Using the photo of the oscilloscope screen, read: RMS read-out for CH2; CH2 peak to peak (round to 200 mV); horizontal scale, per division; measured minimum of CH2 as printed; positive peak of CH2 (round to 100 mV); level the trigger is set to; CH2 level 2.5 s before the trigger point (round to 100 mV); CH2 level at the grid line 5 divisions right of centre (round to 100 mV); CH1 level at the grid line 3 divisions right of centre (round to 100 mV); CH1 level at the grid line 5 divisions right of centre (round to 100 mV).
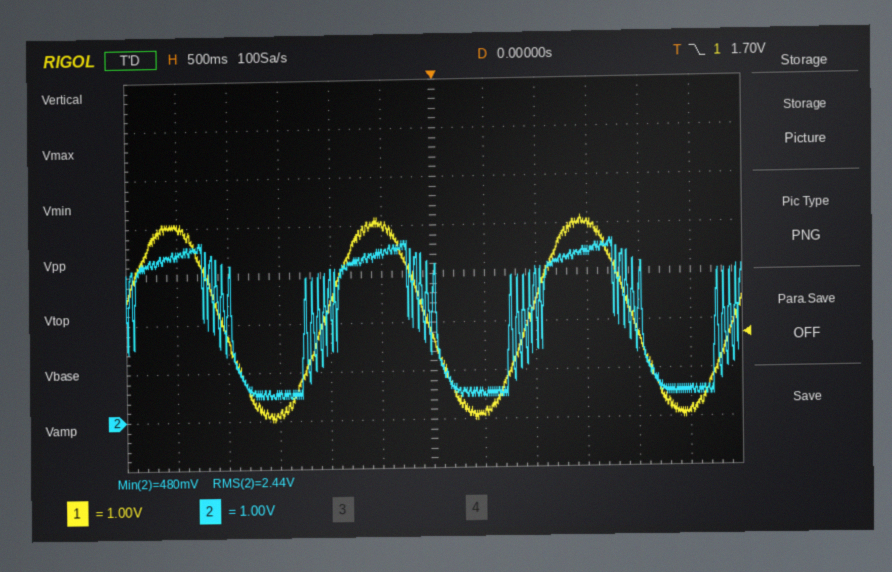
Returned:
2.44 V
3.2 V
500 ms
480 mV
3.7 V
1.70 V
3.4 V
600 mV
4.0 V
200 mV
